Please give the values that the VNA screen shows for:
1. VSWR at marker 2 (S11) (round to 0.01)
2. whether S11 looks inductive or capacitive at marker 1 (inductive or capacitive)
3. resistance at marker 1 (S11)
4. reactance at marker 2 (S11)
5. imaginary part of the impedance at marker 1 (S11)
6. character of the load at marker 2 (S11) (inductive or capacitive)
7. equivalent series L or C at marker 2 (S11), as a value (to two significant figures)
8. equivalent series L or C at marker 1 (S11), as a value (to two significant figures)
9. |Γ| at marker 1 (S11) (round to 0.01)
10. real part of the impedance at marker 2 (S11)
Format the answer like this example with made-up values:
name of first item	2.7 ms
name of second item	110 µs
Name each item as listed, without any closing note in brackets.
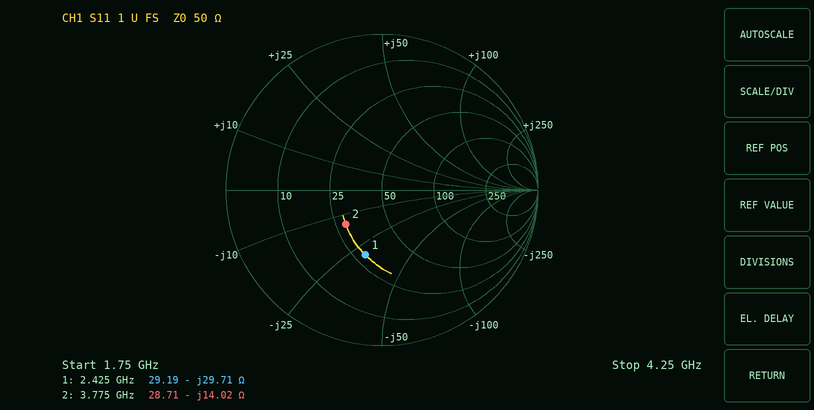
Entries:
VSWR at marker 2 (S11)	1.94
whether S11 looks inductive or capacitive at marker 1	capacitive
resistance at marker 1	29.19 Ω
reactance at marker 2	-14.02 Ω
imaginary part of the impedance at marker 1	-29.71 Ω
character of the load at marker 2 (S11)	capacitive
equivalent series L or C at marker 2 (S11), as a value	3.0 pF
equivalent series L or C at marker 1 (S11), as a value	2.2 pF
|Γ| at marker 1 (S11)	0.43
real part of the impedance at marker 2	28.71 Ω
